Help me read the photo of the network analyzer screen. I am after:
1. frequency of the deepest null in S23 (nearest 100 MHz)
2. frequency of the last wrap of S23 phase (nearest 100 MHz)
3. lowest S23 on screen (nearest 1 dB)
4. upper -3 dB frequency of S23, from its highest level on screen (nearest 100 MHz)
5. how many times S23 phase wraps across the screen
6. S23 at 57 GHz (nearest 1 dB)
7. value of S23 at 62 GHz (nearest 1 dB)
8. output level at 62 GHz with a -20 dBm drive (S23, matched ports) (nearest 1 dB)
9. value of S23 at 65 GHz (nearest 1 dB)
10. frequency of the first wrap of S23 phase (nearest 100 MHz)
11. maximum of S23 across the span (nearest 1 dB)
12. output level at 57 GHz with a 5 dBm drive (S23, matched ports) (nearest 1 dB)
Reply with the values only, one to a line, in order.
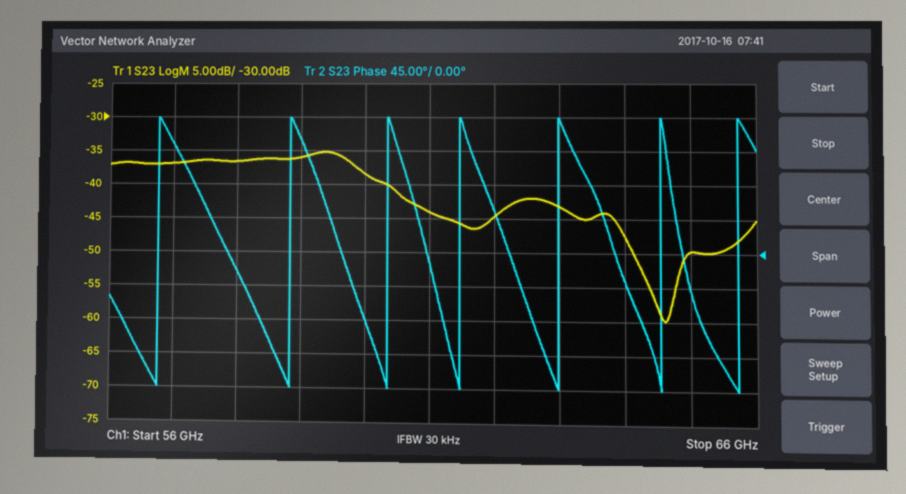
64.6 GHz
65.7 GHz
-60 dB
60.0 GHz
7
-37 dB
-45 dB
-65 dBm
-50 dB
56.8 GHz
-35 dB
-32 dBm
